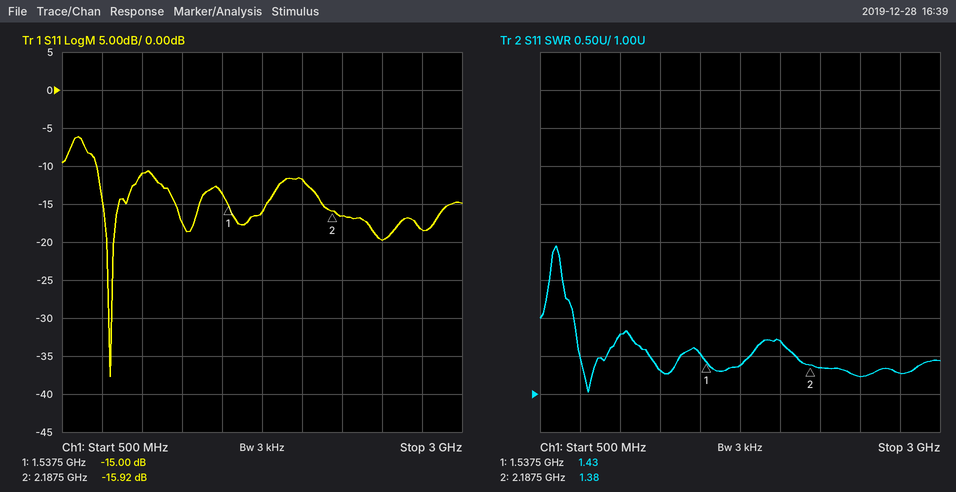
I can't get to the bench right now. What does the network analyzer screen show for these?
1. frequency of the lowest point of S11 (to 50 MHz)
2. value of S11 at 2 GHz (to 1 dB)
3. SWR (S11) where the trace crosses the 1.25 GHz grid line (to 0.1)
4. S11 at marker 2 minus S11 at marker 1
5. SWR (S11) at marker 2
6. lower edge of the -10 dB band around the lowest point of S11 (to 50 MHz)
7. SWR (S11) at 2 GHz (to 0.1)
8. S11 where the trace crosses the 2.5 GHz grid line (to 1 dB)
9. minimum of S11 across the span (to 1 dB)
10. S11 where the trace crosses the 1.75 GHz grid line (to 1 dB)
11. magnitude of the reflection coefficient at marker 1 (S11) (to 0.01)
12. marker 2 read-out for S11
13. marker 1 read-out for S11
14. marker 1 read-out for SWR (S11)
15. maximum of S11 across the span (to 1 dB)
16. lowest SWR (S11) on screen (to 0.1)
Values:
800 MHz
-12 dB
1.3
-0.92 dB
1.38
700 MHz
1.7
-20 dB
-38 dB
-16 dB
0.18
-15.92 dB
-15.00 dB
1.43
-6 dB
1.0
